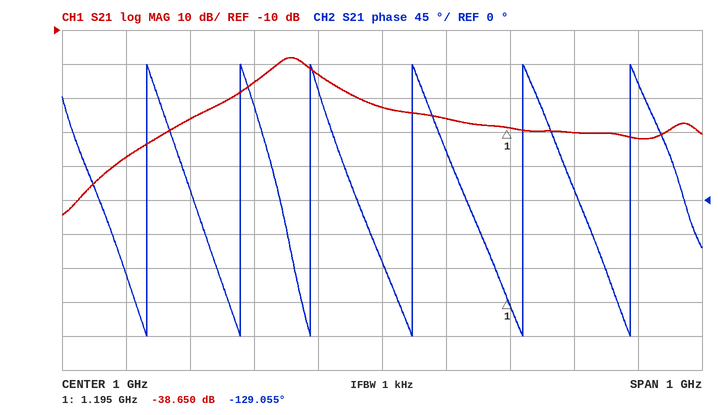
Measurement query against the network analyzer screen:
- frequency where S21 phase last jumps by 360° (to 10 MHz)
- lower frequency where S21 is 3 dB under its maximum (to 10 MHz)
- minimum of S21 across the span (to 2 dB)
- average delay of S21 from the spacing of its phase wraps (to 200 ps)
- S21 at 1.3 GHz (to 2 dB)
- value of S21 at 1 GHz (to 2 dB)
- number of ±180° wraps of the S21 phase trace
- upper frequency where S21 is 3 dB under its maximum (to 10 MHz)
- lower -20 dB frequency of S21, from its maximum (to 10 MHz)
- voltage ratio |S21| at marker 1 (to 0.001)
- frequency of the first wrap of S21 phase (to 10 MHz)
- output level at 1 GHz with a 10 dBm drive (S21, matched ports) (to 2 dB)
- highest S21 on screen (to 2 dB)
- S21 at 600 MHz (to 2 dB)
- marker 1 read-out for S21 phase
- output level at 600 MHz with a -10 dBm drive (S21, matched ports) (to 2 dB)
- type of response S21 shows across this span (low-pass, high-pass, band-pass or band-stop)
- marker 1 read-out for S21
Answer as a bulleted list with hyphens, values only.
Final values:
- 1.39 GHz
- 830 MHz
- -64 dB
- 6.6 ns
- -40 dB
- -32 dB
- 6
- 890 MHz
- 680 MHz
- 0.012
- 630 MHz
- -22 dBm
- -18 dB
- -48 dB
- -129.055°
- -58 dBm
- band-pass
- -38.650 dB
